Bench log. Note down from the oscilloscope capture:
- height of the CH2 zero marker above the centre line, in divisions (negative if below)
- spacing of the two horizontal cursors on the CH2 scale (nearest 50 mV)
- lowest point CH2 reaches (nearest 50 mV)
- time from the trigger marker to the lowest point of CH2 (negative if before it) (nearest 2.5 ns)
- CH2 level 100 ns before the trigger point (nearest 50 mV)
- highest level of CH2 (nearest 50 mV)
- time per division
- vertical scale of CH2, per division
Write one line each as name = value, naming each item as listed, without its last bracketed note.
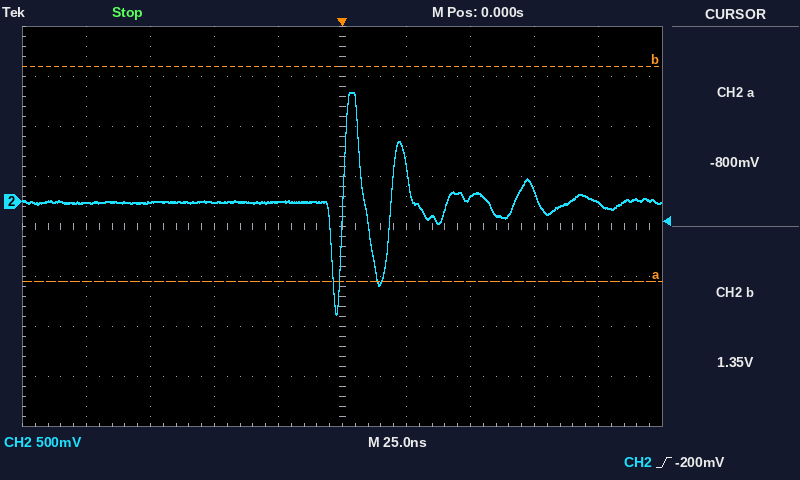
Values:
height of the CH2 zero marker above the centre line, in divisions = +0.5 div
spacing of the two horizontal cursors on the CH2 scale = 2.15 V
lowest point CH2 reaches = -1.15 V
time from the trigger marker to the lowest point of CH2 (negative if before it) = -2.5 ns
CH2 level 100 ns before the trigger point = 0 mV
highest level of CH2 = 1.10 V
time per division = 25 ns
vertical scale of CH2, per division = 500 mV
